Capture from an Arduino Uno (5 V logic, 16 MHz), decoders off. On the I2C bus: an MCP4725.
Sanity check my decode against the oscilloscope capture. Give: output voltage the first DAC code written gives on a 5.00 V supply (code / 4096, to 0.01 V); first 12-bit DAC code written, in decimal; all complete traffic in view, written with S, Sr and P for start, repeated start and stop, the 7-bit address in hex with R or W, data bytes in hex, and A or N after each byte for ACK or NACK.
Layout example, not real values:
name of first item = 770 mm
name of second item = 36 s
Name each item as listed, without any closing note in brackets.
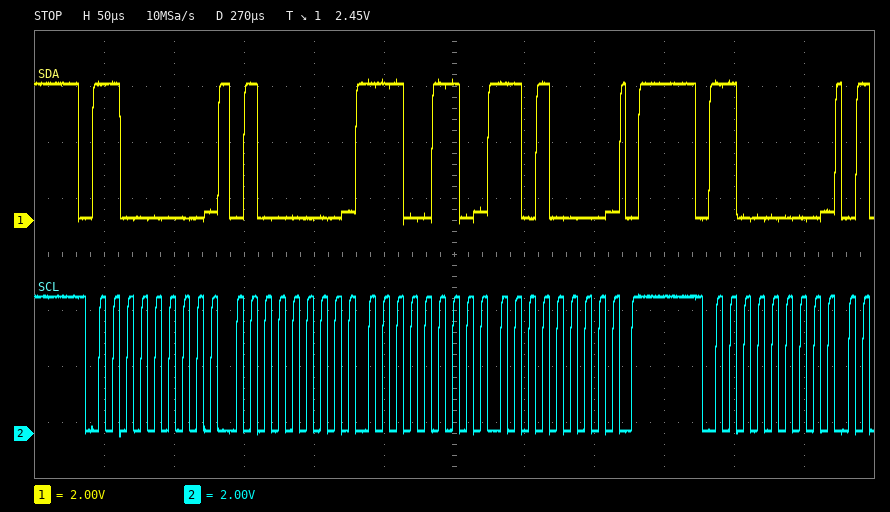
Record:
output voltage the first DAC code written gives on a 5.00 V supply = 4.51 V
first 12-bit DAC code written, in decimal = 3693
all complete traffic in view, written with S, Sr and P for start, repeated start and stop, the 7-bit address in hex with R or W, data bytes in hex, and A or N after each byte for ACK or NACK = S 60W A 40 A E6 A D0 A P S 60W A
